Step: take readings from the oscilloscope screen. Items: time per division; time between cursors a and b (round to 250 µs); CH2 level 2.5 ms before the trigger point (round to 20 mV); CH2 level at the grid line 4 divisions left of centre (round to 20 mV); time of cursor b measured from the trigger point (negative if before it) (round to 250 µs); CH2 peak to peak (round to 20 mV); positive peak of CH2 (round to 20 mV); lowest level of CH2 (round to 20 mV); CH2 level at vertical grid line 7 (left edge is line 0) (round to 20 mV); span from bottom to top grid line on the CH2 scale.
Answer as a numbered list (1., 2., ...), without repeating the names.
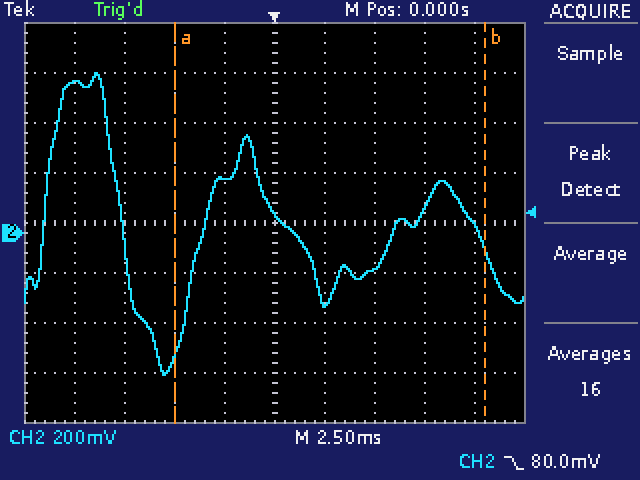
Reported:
1. 2.5 ms
2. 15.50 ms
3. 220 mV
4. 600 mV
5. +10.50 ms
6. 1.20 V
7. 640 mV
8. -560 mV
9. -140 mV
10. 1.6 V
